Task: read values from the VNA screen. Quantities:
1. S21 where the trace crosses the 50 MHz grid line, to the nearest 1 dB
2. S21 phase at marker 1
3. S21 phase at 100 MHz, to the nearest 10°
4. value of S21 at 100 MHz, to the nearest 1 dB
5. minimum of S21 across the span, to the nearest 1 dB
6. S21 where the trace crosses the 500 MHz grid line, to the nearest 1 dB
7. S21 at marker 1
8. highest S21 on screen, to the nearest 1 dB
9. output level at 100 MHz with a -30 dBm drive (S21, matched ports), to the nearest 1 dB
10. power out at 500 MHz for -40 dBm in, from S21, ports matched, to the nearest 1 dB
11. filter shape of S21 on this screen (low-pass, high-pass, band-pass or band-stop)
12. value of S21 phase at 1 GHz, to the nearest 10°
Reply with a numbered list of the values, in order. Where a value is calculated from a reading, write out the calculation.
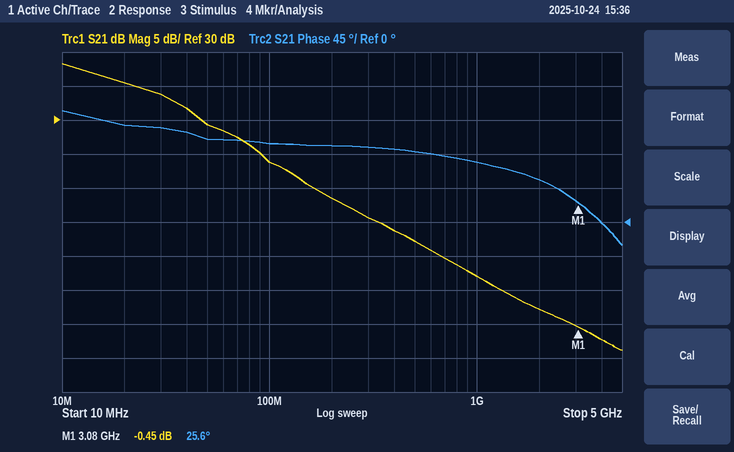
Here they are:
1. 29 dB
2. 25.6°
3. 100°
4. 24 dB
5. -4 dB
6. 12 dB
7. -0.45 dB
8. 38 dB
9. -30 dBm + (24 dB) = -6 dBm
10. -40 dBm + (12 dB) = -28 dBm
11. low-pass
12. 80°
